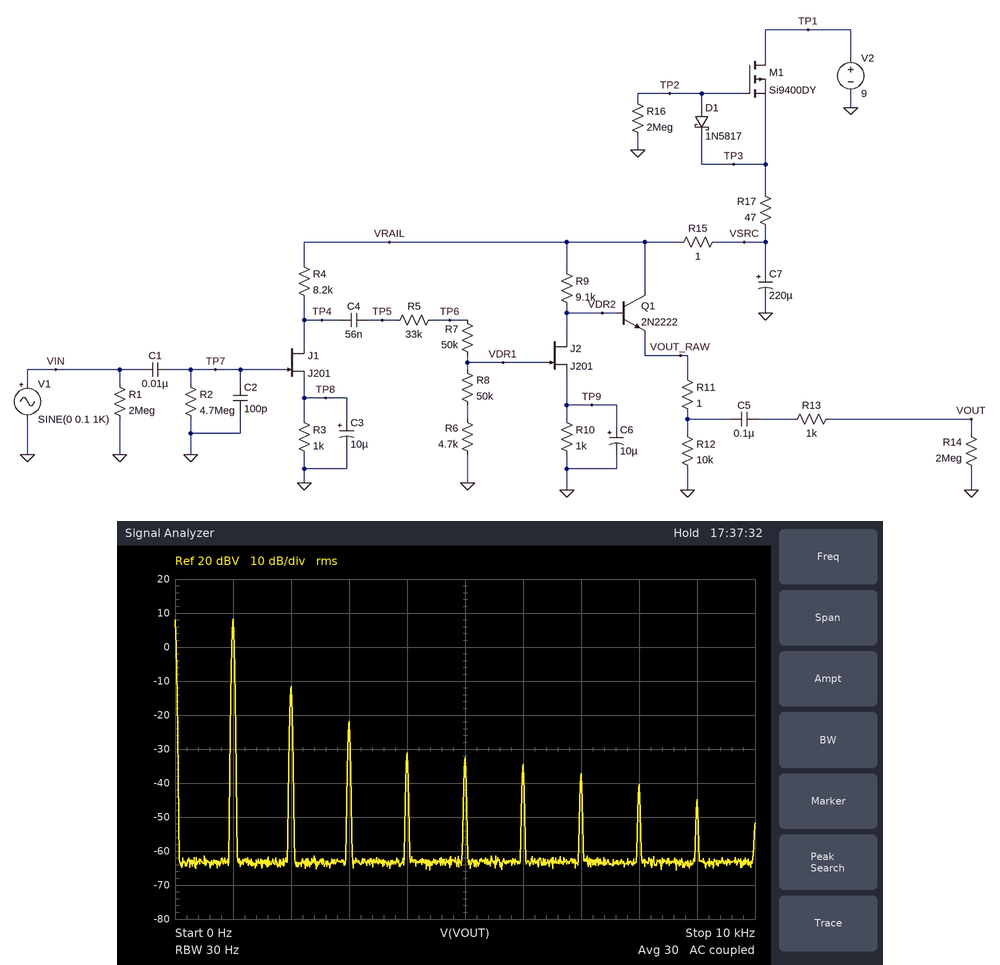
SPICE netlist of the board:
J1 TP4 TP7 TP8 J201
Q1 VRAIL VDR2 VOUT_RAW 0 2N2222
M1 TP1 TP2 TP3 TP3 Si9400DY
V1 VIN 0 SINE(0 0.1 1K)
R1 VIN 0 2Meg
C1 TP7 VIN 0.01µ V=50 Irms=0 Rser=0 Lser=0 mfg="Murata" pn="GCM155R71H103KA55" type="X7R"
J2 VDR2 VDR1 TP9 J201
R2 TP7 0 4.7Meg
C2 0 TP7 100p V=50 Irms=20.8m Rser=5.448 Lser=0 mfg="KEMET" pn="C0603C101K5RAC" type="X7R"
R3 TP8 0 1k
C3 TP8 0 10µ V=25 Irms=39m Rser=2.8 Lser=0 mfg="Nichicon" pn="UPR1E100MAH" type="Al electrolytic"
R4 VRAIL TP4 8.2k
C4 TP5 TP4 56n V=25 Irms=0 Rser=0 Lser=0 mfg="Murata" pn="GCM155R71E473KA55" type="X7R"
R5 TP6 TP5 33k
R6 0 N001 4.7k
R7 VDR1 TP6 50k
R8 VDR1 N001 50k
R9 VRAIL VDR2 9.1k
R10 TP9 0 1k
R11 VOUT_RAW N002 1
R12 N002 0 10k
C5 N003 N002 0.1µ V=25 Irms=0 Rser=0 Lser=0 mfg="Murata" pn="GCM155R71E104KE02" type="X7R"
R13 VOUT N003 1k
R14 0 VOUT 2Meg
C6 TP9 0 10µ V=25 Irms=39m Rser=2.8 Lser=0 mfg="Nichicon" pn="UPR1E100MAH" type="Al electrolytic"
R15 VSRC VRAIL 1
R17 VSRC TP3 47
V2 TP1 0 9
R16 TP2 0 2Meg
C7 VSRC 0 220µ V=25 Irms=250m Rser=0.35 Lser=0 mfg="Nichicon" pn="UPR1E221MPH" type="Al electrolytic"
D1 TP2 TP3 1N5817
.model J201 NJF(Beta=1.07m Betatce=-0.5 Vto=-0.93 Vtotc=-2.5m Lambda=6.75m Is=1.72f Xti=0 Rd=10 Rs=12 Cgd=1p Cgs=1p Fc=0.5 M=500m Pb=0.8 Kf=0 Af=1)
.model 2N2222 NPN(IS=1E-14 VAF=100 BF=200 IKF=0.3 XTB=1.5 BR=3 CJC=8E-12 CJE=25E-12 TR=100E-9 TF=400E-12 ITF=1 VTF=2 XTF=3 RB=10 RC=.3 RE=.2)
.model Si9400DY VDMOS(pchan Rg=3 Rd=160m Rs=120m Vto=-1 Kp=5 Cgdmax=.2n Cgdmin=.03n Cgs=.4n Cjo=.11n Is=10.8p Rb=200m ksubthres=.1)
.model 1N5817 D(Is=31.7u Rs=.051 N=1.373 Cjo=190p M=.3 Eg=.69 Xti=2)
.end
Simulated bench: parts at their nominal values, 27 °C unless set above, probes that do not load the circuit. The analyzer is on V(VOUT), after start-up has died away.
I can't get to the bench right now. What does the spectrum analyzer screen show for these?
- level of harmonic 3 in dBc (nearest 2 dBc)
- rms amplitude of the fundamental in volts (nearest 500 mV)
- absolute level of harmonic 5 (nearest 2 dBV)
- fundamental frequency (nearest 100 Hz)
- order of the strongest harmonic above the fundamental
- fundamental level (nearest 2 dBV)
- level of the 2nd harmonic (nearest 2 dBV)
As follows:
-30 dBc
2.5 V
-32 dBV
1.0 kHz
2
8 dBV
-12 dBV
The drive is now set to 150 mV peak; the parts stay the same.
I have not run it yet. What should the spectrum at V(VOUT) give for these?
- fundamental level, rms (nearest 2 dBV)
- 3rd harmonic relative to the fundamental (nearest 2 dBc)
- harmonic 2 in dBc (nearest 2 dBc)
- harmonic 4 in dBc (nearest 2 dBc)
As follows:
10 dBV
-16 dBc
-24 dBc
-28 dBc
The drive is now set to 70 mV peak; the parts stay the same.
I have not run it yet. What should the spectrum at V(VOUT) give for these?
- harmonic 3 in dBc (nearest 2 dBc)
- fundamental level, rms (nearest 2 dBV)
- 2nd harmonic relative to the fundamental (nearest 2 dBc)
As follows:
-42 dBc
6 dBV
-22 dBc
